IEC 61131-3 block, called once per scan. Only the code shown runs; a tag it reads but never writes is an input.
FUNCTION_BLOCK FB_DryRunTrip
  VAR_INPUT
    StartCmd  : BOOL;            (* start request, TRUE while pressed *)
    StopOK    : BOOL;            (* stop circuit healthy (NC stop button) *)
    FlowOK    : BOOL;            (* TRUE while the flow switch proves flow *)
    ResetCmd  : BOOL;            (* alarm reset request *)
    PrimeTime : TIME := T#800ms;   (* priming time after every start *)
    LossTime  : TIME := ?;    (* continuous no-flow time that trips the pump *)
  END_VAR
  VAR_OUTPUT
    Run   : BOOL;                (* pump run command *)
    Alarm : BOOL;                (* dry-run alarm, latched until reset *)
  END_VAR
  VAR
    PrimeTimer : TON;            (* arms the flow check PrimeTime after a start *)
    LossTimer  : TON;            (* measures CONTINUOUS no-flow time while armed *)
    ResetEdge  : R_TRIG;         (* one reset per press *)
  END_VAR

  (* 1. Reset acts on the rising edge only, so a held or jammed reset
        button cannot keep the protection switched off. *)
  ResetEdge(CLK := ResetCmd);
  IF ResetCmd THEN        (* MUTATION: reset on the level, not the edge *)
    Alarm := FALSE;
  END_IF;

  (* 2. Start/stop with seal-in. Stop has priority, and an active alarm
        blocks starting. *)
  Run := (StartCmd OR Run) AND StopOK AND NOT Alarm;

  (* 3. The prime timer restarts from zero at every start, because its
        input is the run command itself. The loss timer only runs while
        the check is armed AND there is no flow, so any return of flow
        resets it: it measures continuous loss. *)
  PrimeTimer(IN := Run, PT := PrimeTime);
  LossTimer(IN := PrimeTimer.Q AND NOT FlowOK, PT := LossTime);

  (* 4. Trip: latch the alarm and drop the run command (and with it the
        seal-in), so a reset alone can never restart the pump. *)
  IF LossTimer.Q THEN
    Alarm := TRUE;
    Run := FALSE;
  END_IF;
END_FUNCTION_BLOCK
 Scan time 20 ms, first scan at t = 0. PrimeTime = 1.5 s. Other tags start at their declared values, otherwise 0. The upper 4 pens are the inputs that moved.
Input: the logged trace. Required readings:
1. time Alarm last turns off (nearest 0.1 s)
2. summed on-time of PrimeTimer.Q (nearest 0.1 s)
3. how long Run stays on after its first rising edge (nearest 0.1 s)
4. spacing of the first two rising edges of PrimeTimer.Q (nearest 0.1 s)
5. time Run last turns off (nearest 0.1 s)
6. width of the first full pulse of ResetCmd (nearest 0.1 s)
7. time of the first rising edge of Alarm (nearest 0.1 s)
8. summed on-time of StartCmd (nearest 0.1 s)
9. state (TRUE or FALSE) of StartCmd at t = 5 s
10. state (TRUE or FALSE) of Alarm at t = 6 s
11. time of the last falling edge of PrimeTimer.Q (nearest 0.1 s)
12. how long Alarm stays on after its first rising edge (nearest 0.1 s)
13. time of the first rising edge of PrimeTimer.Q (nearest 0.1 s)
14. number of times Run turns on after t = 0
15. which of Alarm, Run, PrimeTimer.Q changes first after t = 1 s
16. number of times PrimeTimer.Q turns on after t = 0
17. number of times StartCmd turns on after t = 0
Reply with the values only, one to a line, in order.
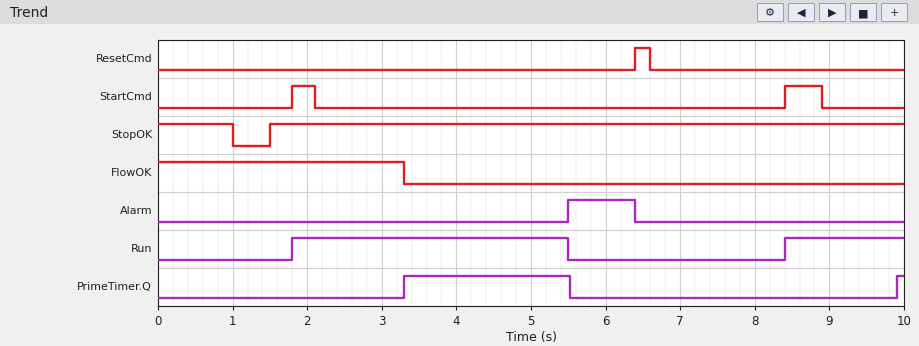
6.4 s
2.3 s
3.7 s
6.6 s
5.5 s
0.2 s
5.5 s
0.8 s
FALSE
TRUE
5.5 s
0.9 s
3.3 s
2
Run
2
2
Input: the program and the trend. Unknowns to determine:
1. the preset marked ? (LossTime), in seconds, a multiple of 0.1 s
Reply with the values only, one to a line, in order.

2.2 s
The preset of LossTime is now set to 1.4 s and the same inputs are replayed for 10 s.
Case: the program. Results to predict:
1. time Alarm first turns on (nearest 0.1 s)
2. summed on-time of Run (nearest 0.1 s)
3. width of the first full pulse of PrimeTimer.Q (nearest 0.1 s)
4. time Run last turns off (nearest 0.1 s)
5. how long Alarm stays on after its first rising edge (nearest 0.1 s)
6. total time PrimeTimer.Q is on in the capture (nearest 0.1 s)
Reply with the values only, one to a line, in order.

4.7 s
4.5 s
1.4 s
4.7 s
1.7 s
1.5 s
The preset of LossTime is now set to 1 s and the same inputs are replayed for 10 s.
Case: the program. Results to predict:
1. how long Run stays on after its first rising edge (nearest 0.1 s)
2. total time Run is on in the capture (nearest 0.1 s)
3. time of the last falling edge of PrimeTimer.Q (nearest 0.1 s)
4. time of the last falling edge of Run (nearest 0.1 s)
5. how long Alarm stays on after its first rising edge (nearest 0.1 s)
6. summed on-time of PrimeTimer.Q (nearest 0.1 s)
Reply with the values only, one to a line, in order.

2.5 s
4.1 s
4.3 s
4.3 s
2.1 s
1.1 s
